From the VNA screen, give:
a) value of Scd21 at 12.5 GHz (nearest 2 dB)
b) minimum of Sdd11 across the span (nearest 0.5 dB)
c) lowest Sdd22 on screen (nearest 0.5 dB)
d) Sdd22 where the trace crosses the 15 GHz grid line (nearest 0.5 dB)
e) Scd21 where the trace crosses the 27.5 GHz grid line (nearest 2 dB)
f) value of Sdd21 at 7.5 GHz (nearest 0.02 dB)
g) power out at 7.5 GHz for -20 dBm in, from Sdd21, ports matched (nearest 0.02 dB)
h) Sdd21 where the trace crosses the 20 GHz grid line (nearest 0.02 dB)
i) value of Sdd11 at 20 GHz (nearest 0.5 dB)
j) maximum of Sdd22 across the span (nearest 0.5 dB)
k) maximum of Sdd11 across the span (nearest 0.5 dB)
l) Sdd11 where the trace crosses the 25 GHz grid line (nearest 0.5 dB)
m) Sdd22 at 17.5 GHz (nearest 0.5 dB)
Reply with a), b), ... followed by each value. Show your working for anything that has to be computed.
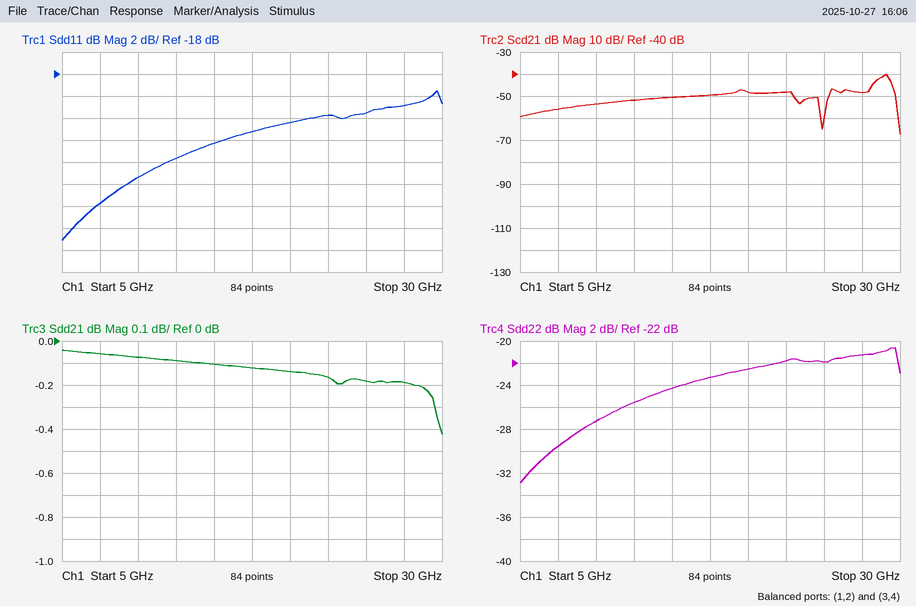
a) -52 dB
b) -33.0 dB
c) -33.0 dB
d) -24.5 dB
e) -48 dB
f) -0.06 dB
g) -20 dBm + (-0.06 dB) = -20.06 dBm
h) -0.14 dB
i) -22.5 dB
j) -20.5 dB
k) -19.5 dB
l) -21.5 dB
m) -23.5 dB
